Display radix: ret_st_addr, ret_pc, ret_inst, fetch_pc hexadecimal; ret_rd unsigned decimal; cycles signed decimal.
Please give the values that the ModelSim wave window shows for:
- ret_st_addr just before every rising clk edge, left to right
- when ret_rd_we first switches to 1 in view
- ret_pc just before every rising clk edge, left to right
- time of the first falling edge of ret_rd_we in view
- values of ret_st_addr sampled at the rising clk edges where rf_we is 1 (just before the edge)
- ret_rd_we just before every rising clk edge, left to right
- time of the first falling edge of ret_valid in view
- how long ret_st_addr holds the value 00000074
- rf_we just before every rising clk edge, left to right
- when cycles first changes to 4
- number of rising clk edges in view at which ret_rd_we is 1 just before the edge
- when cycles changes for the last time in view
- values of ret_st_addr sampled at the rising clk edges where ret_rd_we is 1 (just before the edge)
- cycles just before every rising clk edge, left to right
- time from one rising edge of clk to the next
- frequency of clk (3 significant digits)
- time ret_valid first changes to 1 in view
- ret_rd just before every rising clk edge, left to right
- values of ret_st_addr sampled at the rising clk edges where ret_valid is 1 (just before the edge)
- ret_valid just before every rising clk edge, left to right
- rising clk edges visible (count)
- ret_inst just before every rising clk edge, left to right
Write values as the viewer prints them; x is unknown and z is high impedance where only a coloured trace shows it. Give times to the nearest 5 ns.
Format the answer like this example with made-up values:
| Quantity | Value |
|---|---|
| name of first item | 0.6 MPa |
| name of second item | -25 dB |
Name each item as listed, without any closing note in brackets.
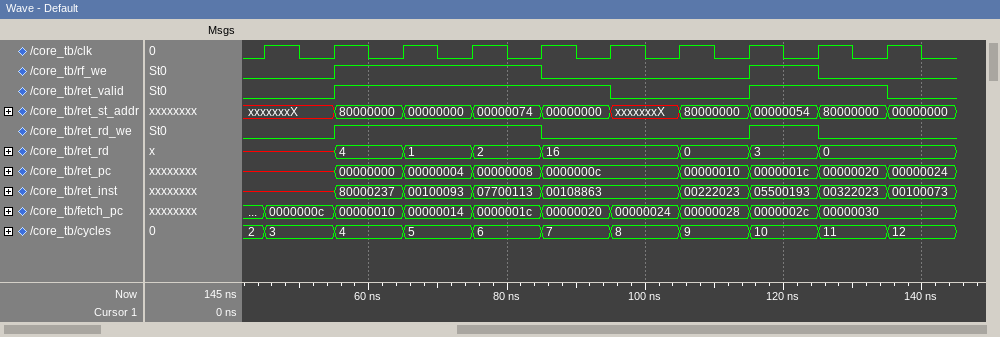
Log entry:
| Quantity | Value |
|---|---|
| ret_st_addr just before every rising clk edge, left to right | xxxxxxxX, xxxxxxxX, 80000000, 00000000, 00000074, 00000000, xxxxxxxX, 80000000, 00000054, 80000000 |
| when ret_rd_we first switches to 1 in view | 55 ns |
| ret_pc just before every rising clk edge, left to right | x, x, 00000000, 00000004, 00000008, 0000000c, 0000000c, 00000010, 0000001c, 00000020 |
| time of the first falling edge of ret_rd_we in view | 85 ns |
| values of ret_st_addr sampled at the rising clk edges where rf_we is 1 | 80000000, 00000000, 00000074, 00000054 |
| ret_rd_we just before every rising clk edge, left to right | 0 0 1 1 1 0 0 0 1 0 |
| time of the first falling edge of ret_valid in view | 95 ns |
| how long ret_st_addr holds the value 00000074 | 10 ns |
| rf_we just before every rising clk edge, left to right | 0 0 1 1 1 0 0 0 1 0 |
| when cycles first changes to 4 | 55 ns |
| number of rising clk edges in view at which ret_rd_we is 1 just before the edge | 4 |
| when cycles changes for the last time in view | 135 ns |
| values of ret_st_addr sampled at the rising clk edges where ret_rd_we is 1 | 80000000, 00000000, 00000074, 00000054 |
| cycles just before every rising clk edge, left to right | 2, 3, 4, 5, 6, 7, 8, 9, 10, 11 |
| time from one rising edge of clk to the next | 10 ns |
| frequency of clk | 100 MHz |
| time ret_valid first changes to 1 in view | 55 ns |
| ret_rd just before every rising clk edge, left to right | x, x, 4, 1, 2, 16, 16, 0, 3, 0 |
| values of ret_st_addr sampled at the rising clk edges where ret_valid is 1 | 80000000, 00000000, 00000074, 00000000, 00000054, 80000000 |
| ret_valid just before every rising clk edge, left to right | 0 0 1 1 1 1 0 0 1 1 |
| rising clk edges visible | 10 |
| ret_inst just before every rising clk edge, left to right | x, x, 80000237, 00100093, 07700113, 00108863, 00108863, 00222023, 05500193, 00322023 |
